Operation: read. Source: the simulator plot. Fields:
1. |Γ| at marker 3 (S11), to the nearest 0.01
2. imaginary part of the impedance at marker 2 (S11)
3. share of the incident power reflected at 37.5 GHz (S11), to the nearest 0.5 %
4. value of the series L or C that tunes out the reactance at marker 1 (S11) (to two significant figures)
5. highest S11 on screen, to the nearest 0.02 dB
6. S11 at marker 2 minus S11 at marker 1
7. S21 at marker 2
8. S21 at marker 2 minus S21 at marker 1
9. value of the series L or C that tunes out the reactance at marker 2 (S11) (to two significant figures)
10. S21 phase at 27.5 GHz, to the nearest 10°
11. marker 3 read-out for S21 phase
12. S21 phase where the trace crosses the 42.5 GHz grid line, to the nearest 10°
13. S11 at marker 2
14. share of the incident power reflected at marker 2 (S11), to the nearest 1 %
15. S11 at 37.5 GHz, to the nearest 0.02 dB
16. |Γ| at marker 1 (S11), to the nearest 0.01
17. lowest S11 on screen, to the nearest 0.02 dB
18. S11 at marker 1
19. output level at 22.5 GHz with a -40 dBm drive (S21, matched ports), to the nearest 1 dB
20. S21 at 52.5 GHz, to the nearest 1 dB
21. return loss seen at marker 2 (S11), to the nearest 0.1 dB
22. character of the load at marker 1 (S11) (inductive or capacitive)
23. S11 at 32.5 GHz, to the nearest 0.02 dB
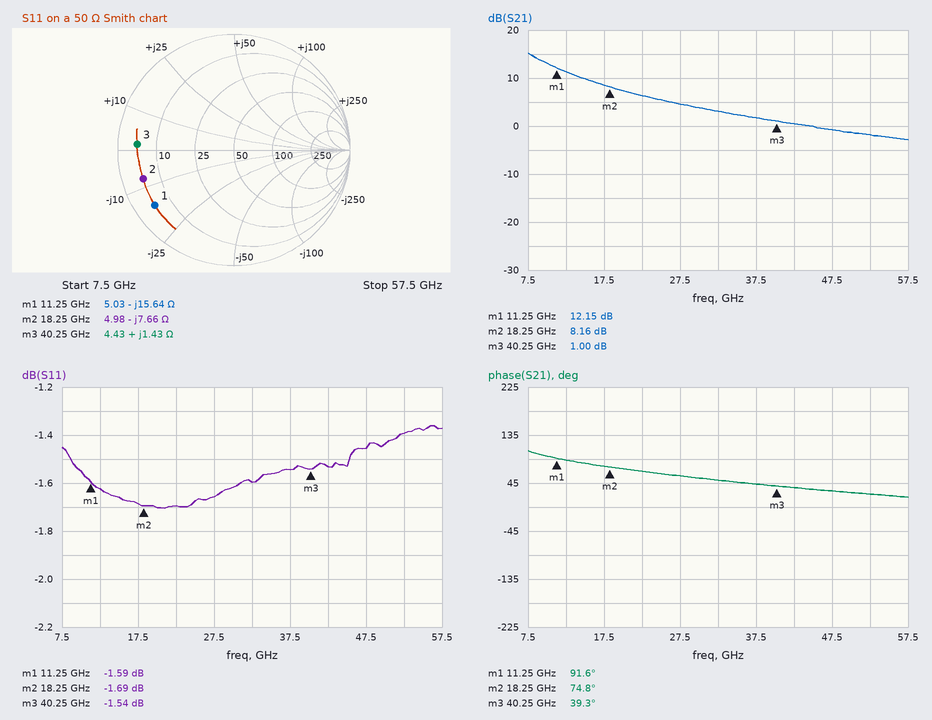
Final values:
0.84
-7.66 Ω
70.0 %
220 pH
-1.36 dB
-0.10 dB
8.16 dB
-3.99 dB
67 pH
60°
39.3°
40°
-1.69 dB
68 %
-1.54 dB
0.83
-1.70 dB
-1.59 dB
-34 dBm
-2 dB
1.7 dB
capacitive
-1.60 dB
